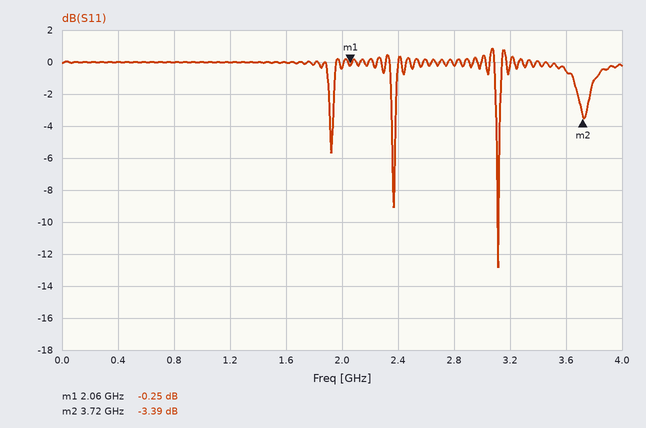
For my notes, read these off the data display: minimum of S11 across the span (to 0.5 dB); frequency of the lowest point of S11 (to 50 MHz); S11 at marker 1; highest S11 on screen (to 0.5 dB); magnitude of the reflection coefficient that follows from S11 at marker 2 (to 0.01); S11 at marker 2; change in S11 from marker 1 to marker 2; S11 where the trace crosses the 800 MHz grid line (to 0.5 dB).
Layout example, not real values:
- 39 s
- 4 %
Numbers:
- -13.0 dB
- 3.10 GHz
- -0.25 dB
- 1.0 dB
- 0.68
- -3.39 dB
- -3.14 dB
- 0.0 dB
